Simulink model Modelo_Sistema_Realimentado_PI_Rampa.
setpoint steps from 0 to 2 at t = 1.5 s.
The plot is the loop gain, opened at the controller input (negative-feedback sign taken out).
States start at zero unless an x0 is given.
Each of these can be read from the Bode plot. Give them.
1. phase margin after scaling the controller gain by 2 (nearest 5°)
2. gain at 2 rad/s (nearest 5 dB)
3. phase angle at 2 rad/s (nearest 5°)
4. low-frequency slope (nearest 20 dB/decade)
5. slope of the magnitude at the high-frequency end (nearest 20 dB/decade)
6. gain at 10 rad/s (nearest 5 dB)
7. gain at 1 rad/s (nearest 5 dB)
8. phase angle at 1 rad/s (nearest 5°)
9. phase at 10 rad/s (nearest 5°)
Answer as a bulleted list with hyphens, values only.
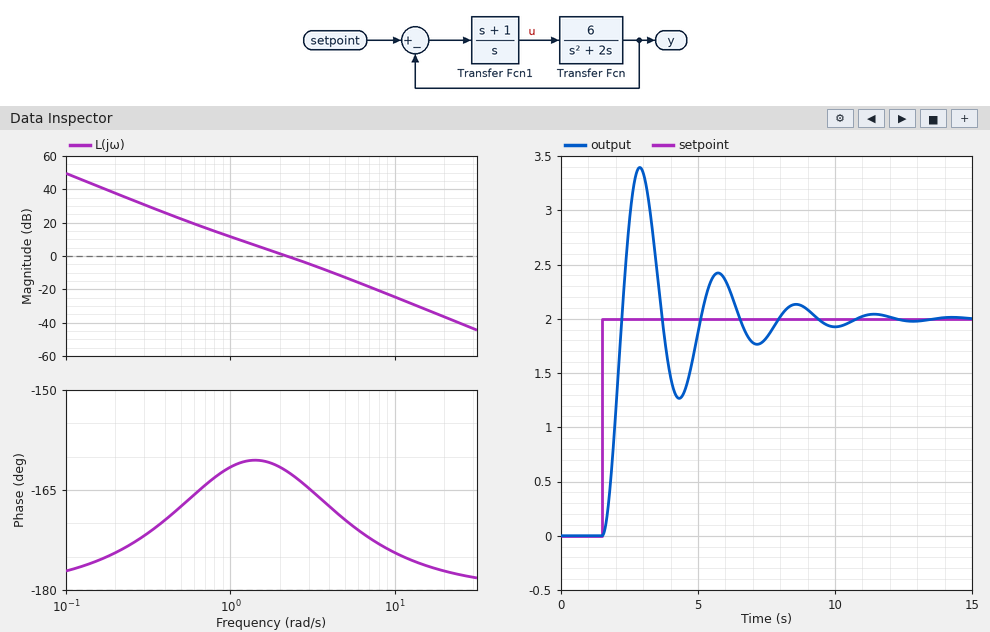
- 15°
- 0 dB
- -160°
- -40 dB/decade
- -40 dB/decade
- -25 dB
- 10 dB
- -160°
- -175°
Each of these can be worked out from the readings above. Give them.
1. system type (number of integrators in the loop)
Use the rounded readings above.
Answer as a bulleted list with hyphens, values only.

- 2
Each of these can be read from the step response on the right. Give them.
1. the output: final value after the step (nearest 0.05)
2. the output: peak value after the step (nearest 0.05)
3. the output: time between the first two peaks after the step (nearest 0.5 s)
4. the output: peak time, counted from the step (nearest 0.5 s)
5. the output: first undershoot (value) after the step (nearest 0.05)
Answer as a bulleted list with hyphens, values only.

- 2.00
- 3.40
- 3.0 s
- 1.5 s
- 1.25
